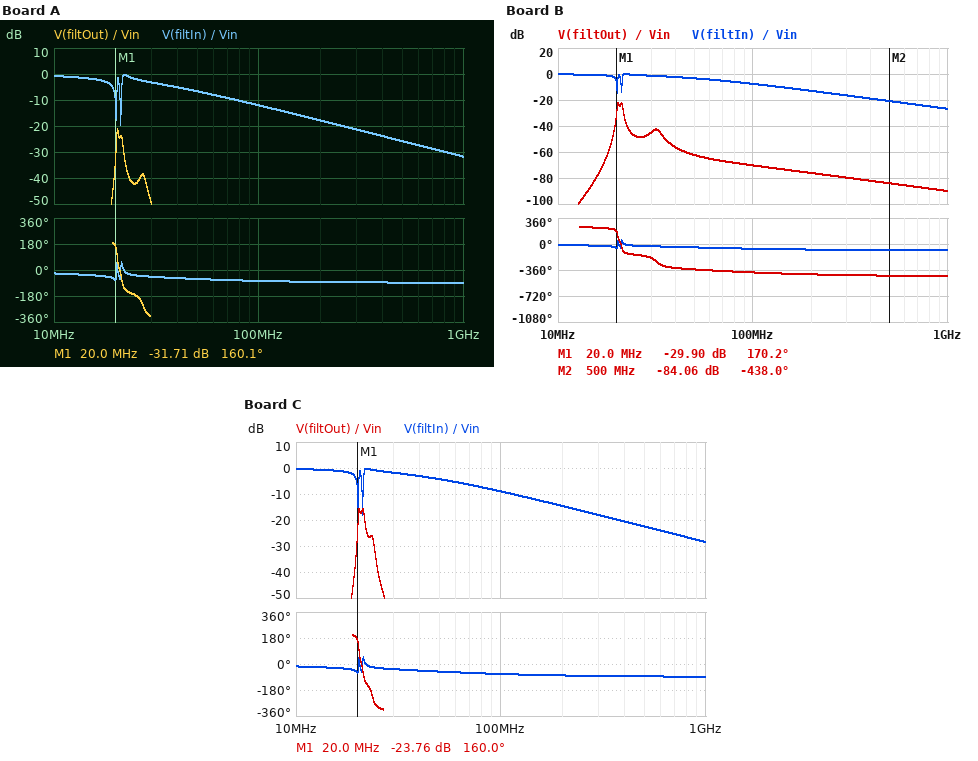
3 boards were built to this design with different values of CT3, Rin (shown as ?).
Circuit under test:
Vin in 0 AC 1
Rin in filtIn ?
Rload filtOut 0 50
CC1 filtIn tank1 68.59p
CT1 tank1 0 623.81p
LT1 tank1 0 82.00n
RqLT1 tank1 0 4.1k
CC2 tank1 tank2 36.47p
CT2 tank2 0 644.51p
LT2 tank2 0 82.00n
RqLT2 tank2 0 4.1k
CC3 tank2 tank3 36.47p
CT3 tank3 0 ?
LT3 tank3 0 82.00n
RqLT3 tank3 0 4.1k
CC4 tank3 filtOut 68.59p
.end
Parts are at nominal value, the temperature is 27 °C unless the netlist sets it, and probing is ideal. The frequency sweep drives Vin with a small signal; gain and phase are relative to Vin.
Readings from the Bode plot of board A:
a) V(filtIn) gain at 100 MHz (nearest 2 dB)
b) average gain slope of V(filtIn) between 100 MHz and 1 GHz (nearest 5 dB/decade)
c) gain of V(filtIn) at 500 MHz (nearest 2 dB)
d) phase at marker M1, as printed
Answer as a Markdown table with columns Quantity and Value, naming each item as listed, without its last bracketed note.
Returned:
| Quantity | Value |
|---|---|
| V(filtIn) gain at 100 MHz | -12 dB |
| average gain slope of V(filtIn) between 100 MHz and 1 GHz | -20 dB/decade |
| gain of V(filtIn) at 500 MHz | -26 dB |
| phase at marker M1, as printed | 160.1 deg |
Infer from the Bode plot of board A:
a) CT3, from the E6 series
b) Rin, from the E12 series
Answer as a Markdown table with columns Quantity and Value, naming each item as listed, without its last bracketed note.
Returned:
| Quantity | Value |
|---|---|
| CT3, from the E6 series | 330 pF |
| Rin, from the E12 series | 100 Ω |
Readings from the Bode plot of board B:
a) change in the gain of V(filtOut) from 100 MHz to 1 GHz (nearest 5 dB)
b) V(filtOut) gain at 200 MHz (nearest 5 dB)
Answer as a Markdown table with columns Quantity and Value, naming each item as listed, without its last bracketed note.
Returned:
| Quantity | Value |
|---|---|
| change in the gain of V(filtOut) from 100 MHz to 1 GHz | -20 dB |
| V(filtOut) gain at 200 MHz | -75 dB |
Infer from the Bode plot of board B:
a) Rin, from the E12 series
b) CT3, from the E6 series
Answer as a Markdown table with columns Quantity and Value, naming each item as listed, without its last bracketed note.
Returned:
| Quantity | Value |
|---|---|
| Rin, from the E12 series | 56 Ω |
| CT3, from the E6 series | 220 pF |
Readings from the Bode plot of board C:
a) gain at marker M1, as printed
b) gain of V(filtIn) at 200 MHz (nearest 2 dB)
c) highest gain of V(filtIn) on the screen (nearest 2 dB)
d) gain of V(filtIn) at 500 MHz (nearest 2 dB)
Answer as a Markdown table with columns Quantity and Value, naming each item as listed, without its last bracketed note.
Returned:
| Quantity | Value |
|---|---|
| gain at marker M1, as printed | -23.76 dB |
| gain of V(filtIn) at 200 MHz | -14 dB |
| highest gain of V(filtIn) on the screen | 0 dB |
| gain of V(filtIn) at 500 MHz | -22 dB |
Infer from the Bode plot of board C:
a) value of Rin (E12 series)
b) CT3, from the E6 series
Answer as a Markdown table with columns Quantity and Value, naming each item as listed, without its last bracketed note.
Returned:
| Quantity | Value |
|---|---|
| value of Rin | 68 Ω |
| CT3, from the E6 series | 470 pF |
